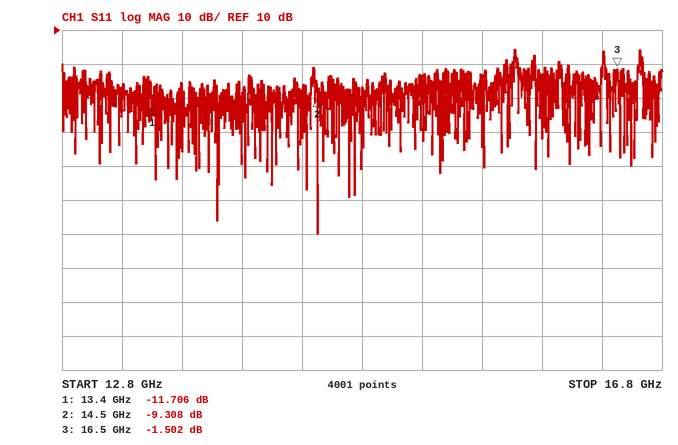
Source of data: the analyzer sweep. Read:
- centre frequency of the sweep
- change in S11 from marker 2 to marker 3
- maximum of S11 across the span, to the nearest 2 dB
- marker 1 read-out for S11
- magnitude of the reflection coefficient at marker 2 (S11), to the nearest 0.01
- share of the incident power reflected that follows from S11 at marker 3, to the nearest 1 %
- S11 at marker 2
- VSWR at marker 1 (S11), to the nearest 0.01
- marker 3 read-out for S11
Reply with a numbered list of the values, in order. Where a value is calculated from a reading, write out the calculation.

1. 14.8 GHz
2. -1.502 − (-9.308) = 7.806 dB
3. 4 dB
4. -11.706 dB
5. 10^(-9.308/20) ≈ 0.34
6. 10^(-1.502/10) ≈ 71 %
7. -9.308 dB
8. (1 + 0.2598)/(1 − 0.2598) ≈ 1.70
9. -1.502 dB
